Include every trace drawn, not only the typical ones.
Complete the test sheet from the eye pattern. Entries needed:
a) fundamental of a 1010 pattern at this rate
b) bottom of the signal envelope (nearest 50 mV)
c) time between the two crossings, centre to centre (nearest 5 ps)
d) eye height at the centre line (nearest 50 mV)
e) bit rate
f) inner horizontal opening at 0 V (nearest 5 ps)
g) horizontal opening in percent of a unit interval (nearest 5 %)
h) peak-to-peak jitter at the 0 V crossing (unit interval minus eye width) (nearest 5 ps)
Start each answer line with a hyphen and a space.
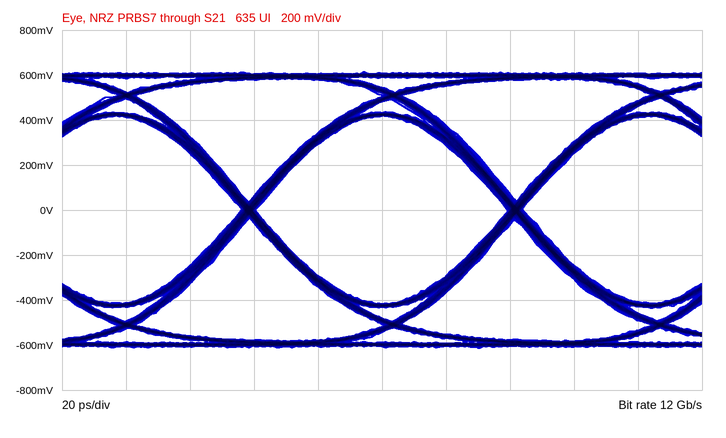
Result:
- 6 GHz
- -600 mV
- 85 ps
- 850 mV
- 12 Gb/s
- 80 ps
- 95 %
- 5 ps
